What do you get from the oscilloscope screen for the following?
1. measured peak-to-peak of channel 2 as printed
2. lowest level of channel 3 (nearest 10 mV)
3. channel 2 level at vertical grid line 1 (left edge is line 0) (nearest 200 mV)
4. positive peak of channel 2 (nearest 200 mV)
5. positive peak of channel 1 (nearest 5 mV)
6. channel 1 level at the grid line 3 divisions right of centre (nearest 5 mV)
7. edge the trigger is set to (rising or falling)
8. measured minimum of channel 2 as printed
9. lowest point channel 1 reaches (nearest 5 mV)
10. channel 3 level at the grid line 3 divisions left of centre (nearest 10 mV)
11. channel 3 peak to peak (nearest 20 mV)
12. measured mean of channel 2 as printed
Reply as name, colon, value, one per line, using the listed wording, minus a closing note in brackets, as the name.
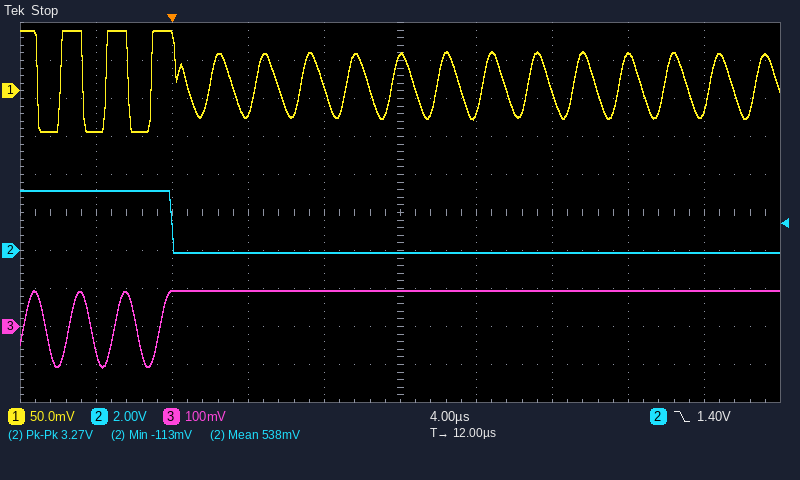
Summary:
measured peak-to-peak of channel 2 as printed: 3.27 V
lowest level of channel 3: -110 mV
channel 2 level at vertical grid line 1 (left edge is line 0): 3.2 V
positive peak of channel 2: 3.2 V
positive peak of channel 1: 80 mV
channel 1 level at the grid line 3 divisions right of centre: 45 mV
edge the trigger is set to: falling
measured minimum of channel 2 as printed: -113 mV
lowest point channel 1 reaches: -55 mV
channel 3 level at the grid line 3 divisions left of centre: 90 mV
channel 3 peak to peak: 200 mV
measured mean of channel 2 as printed: 538 mV
